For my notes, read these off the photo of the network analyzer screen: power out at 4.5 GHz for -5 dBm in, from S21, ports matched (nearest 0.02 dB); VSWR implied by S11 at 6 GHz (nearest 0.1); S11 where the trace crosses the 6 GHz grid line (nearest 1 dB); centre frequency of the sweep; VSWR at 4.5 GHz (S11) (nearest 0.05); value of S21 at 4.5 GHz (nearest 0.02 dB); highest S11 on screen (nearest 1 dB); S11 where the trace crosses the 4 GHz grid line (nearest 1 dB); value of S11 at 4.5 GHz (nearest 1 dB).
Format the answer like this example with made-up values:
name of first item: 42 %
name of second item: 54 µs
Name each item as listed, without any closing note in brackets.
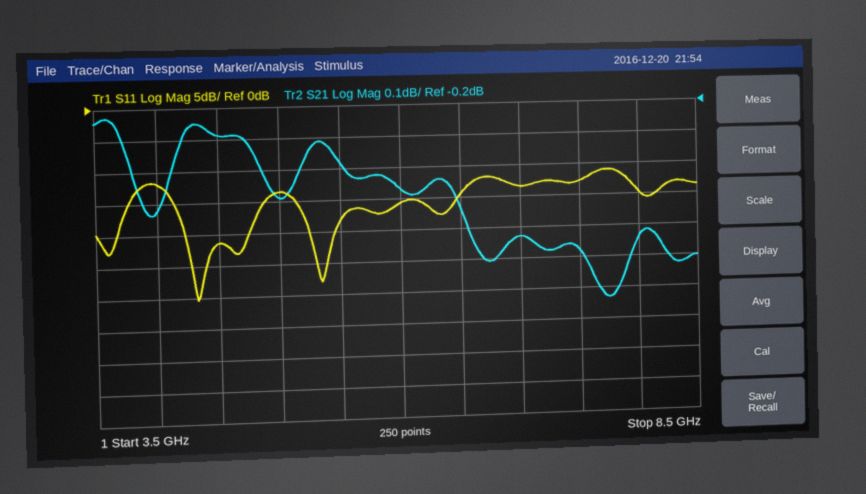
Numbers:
power out at 4.5 GHz for -5 dBm in, from S21, ports matched: -5.28 dBm
VSWR implied by S11 at 6 GHz: 1.4
S11 where the trace crosses the 6 GHz grid line: -16 dB
centre frequency of the sweep: 6 GHz
VSWR at 4.5 GHz (S11): 1.20
value of S21 at 4.5 GHz: -0.28 dB
highest S11 on screen: -11 dB
S11 where the trace crosses the 4 GHz grid line: -12 dB
value of S11 at 4.5 GHz: -21 dB
